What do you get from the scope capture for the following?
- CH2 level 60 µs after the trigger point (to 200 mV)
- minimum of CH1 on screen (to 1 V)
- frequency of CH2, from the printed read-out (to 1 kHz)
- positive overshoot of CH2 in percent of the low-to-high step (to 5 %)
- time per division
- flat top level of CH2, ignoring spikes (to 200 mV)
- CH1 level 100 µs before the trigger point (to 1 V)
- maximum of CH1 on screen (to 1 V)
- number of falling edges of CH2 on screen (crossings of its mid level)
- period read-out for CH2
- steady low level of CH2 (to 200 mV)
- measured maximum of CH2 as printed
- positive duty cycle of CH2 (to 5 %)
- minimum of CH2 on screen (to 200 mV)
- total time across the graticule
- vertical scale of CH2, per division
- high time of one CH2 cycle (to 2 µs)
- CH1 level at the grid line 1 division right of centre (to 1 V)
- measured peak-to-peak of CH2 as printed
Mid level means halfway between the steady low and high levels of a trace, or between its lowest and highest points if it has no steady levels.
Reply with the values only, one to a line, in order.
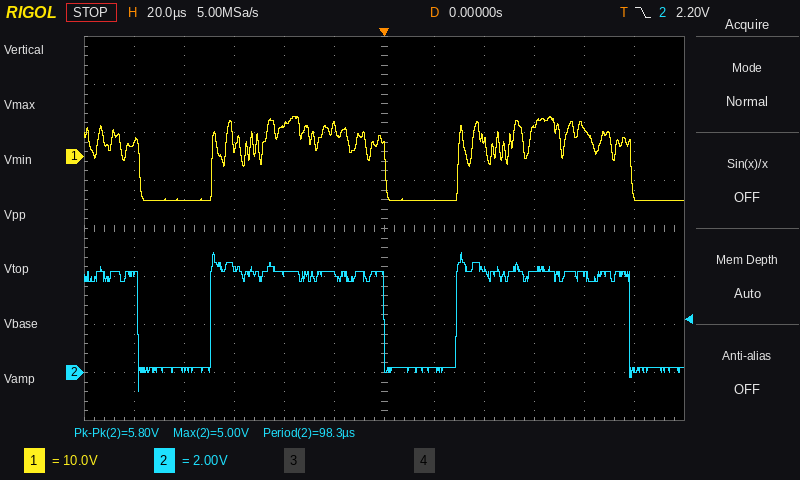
4.2 V
-9 V
10 kHz
20 %
20 µs
4.2 V
3 V
8 V
3
98.3 µs
200 mV
5.00 V
70 %
-800 mV
240 µs
2 V
70 µs
-9 V
5.80 V
